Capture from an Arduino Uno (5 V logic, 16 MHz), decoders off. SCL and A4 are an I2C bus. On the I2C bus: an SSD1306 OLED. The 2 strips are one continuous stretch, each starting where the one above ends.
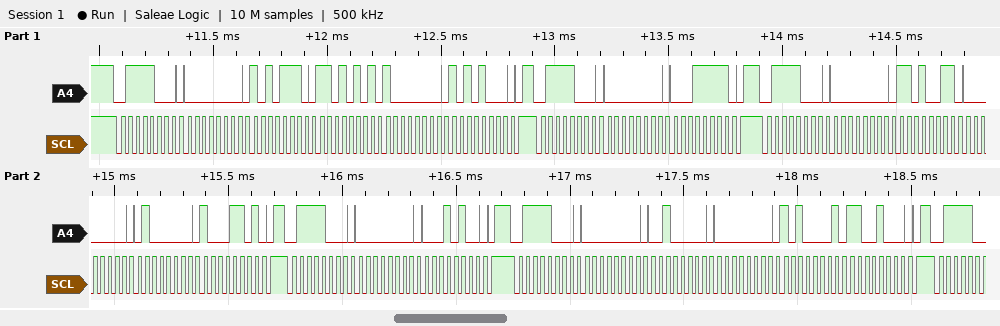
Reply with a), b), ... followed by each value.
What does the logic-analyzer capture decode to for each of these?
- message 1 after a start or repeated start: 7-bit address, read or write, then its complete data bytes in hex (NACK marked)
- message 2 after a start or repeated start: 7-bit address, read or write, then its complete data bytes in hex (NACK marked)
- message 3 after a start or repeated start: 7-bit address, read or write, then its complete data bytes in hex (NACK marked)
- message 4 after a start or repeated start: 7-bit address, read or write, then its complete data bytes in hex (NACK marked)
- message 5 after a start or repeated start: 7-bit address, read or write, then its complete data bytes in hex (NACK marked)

a) 0x3C write: 00 AE D5 80 A8
b) 0x3C write: 00 1F
c) 0x3C write: 00 D3 00 40 8D
d) 0x3C write: 00 14
e) 0x3C write: 00 20 00 A1 C8
